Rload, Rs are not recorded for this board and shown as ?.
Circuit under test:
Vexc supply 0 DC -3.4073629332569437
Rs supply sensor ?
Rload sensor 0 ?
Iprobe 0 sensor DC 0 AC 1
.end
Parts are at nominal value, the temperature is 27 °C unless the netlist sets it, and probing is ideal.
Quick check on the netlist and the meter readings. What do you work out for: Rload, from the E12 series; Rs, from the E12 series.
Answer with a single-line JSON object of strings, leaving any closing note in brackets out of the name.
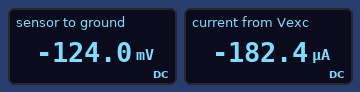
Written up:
{"Rload, from the E12 series": "680 Ω", "Rs, from the E12 series": "18 kΩ"}
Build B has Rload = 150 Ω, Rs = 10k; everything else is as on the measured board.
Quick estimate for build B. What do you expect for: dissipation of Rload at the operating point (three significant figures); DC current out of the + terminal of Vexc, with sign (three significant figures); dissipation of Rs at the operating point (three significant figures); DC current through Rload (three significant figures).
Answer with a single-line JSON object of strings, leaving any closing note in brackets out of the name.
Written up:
{"dissipation of Rload at the operating point": "16.9 µW", "DC current out of the + terminal of Vexc, with sign": "-336 µA", "dissipation of Rs at the operating point": "1.13 mW", "DC current through Rload": "336 µA"}
